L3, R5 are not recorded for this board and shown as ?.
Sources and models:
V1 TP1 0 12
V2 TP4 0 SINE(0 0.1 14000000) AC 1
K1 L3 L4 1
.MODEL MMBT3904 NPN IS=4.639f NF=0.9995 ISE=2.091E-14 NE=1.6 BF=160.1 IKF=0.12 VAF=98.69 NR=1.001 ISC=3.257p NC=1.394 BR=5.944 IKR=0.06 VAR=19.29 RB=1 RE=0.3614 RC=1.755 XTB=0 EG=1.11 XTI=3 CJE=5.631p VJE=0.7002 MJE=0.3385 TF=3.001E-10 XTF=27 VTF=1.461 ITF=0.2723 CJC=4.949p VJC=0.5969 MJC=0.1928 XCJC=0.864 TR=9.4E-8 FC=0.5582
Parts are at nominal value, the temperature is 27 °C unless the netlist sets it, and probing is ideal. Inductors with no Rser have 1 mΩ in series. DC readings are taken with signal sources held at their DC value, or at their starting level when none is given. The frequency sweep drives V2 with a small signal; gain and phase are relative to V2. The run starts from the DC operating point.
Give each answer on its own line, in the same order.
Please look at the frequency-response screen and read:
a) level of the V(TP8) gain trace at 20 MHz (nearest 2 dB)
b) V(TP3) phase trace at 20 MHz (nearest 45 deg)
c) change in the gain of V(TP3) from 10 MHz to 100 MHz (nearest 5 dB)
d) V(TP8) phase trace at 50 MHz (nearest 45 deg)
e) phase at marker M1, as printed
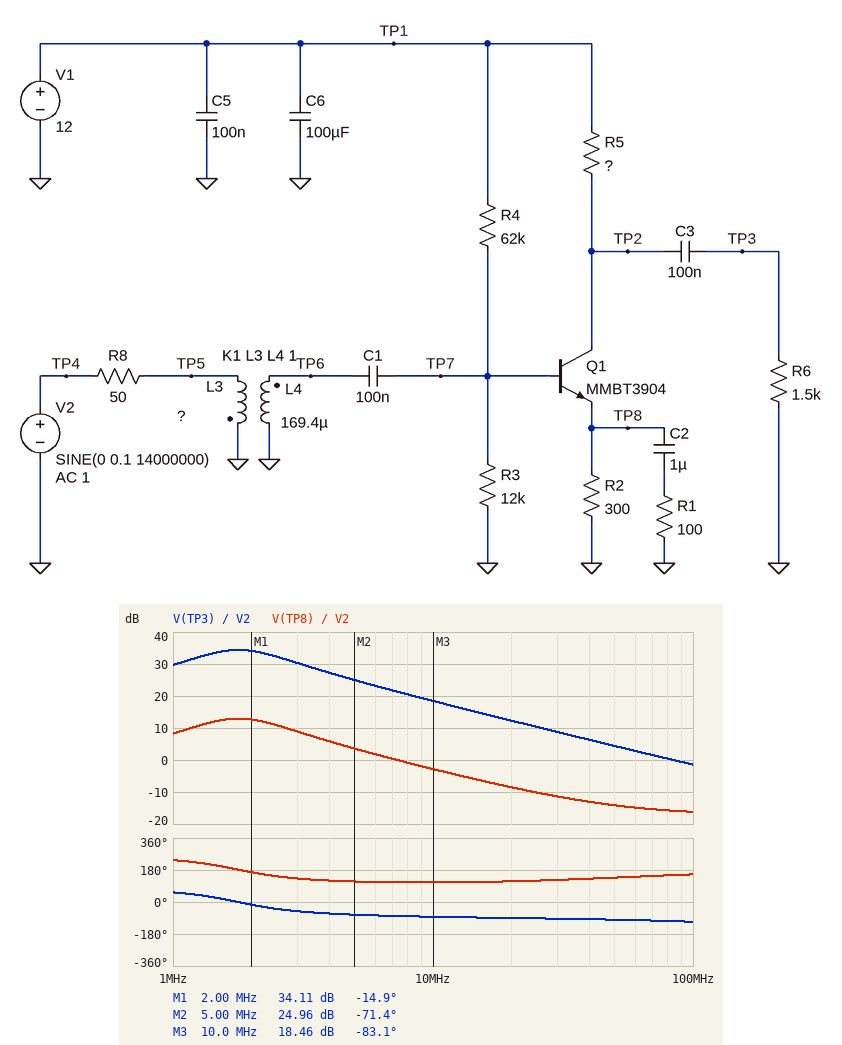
-8 dB
-90 deg
-20 dB
135 deg
-14.9 deg
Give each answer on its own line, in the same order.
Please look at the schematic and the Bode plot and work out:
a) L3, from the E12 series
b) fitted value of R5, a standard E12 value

2.2 µH
2.2 kΩ
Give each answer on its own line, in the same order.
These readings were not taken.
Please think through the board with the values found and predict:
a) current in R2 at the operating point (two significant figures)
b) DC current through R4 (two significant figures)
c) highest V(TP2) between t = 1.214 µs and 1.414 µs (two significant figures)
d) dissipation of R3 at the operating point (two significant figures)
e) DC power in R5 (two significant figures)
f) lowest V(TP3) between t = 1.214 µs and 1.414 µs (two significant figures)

3.4 mA
170 µA
5.2 V
250 µW
25 mW
-590 mV
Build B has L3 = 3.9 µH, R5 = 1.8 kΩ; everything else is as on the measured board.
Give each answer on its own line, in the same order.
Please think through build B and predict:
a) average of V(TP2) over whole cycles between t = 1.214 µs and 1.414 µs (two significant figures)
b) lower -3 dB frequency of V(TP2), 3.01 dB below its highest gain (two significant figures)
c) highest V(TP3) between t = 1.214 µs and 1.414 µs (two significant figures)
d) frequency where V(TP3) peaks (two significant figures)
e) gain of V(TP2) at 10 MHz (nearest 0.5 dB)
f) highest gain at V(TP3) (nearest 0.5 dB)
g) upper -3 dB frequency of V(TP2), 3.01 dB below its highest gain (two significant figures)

5.9 V
1.0 MHz
800 mV
1.9 MHz
21.0 dB
33.0 dB
3.5 MHz
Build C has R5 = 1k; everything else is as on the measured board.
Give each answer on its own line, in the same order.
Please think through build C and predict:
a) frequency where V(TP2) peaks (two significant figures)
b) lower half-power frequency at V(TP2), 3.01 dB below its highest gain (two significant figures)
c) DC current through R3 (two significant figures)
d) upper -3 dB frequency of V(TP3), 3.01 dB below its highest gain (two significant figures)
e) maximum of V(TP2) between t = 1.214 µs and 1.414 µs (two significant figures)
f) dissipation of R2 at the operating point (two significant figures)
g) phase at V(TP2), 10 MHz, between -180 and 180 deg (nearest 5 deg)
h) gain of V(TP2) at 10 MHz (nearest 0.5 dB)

2.2 MHz
1.3 MHz
140 µA
3.7 MHz
9.2 V
3.5 mW
-80 deg
19.0 dB
